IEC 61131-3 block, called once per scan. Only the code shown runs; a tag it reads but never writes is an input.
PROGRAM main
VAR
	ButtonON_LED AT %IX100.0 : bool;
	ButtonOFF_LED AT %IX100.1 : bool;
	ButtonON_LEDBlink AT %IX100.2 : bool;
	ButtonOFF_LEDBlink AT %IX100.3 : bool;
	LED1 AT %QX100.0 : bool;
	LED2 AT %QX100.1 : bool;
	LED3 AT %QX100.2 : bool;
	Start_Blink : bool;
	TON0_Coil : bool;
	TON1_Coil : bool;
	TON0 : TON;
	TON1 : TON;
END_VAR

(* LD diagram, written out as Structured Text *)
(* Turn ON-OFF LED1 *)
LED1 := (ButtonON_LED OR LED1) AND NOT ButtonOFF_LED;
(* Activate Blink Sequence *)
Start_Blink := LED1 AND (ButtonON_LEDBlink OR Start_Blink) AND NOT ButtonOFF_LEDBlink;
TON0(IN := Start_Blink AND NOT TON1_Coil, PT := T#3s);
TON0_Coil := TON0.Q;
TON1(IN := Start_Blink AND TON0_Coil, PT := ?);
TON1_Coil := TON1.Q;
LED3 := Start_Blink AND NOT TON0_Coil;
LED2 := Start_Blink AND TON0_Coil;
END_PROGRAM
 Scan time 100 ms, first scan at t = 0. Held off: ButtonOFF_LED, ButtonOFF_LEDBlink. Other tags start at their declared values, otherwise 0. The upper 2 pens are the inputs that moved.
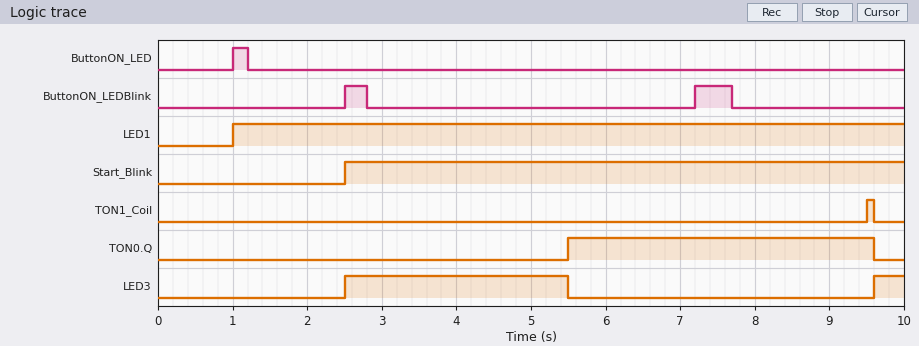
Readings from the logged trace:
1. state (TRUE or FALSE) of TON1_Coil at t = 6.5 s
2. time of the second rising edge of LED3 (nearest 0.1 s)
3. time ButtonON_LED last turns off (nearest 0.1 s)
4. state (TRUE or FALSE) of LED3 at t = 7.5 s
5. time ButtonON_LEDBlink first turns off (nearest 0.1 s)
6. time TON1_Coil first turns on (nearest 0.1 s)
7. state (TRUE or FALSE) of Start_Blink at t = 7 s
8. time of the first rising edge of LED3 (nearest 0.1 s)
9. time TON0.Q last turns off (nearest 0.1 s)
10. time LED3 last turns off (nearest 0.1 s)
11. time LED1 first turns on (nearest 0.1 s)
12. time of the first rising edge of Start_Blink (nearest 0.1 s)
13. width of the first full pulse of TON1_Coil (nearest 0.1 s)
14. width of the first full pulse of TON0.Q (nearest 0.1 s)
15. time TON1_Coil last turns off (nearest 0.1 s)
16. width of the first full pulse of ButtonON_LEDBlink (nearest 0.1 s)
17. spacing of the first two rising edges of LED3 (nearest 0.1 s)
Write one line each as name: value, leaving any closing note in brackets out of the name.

state (TRUE or FALSE) of TON1_Coil at t = 6.5 s: FALSE
time of the second rising edge of LED3: 9.6 s
time ButtonON_LED last turns off: 1.2 s
state (TRUE or FALSE) of LED3 at t = 7.5 s: FALSE
time ButtonON_LEDBlink first turns off: 2.8 s
time TON1_Coil first turns on: 9.5 s
state (TRUE or FALSE) of Start_Blink at t = 7 s: TRUE
time of the first rising edge of LED3: 2.5 s
time TON0.Q last turns off: 9.6 s
time LED3 last turns off: 5.5 s
time LED1 first turns on: 1.0 s
time of the first rising edge of Start_Blink: 2.5 s
width of the first full pulse of TON1_Coil: 0.1 s
width of the first full pulse of TON0.Q: 4.1 s
time TON1_Coil last turns off: 9.6 s
width of the first full pulse of ButtonON_LEDBlink: 0.3 s
spacing of the first two rising edges of LED3: 7.1 s
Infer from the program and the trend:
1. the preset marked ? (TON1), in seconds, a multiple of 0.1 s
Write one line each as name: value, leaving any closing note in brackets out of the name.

the preset marked ? (TON1), in seconds, a multiple of 0.1 s: 4.0 s
